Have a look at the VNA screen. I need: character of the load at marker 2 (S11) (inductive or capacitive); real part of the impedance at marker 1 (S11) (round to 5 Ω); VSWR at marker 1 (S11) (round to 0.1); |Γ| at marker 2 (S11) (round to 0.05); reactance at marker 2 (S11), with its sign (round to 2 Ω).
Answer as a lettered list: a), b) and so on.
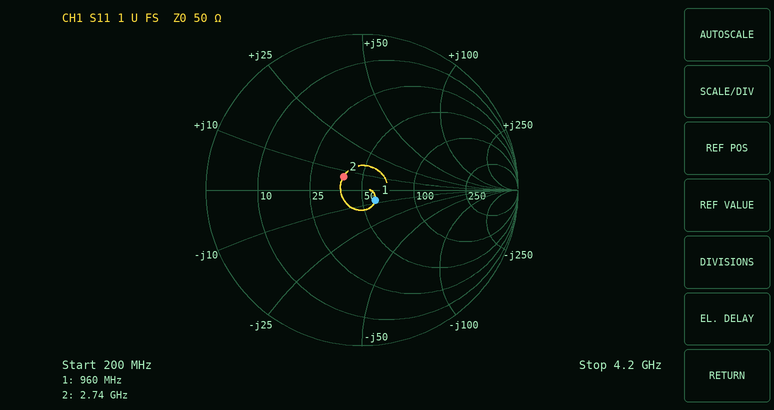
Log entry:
a) inductive
b) 60 Ω
c) 1.2
d) 0.15
e) +6 Ω
